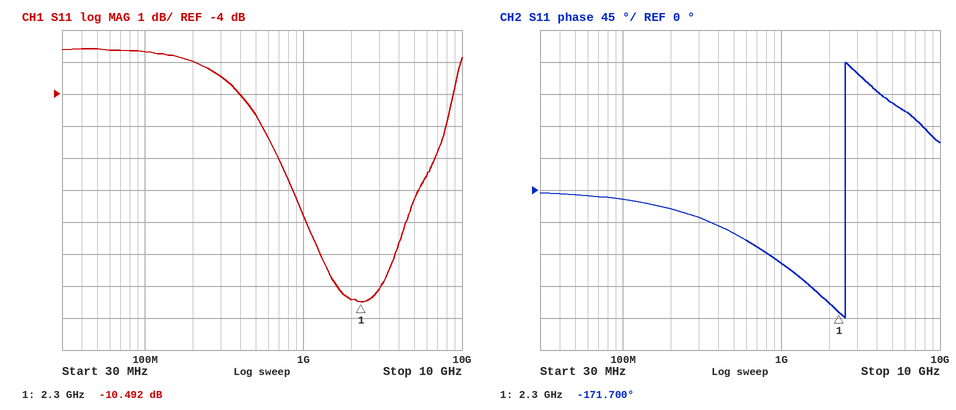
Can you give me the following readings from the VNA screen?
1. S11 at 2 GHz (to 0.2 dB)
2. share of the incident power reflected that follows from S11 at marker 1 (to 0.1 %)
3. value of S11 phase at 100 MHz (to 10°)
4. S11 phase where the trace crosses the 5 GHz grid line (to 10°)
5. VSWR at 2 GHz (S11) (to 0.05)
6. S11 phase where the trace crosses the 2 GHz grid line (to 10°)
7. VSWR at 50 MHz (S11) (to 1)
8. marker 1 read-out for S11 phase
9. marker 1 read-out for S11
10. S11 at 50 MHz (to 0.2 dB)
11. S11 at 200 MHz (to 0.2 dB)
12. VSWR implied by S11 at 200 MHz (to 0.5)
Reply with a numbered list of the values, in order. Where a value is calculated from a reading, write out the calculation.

1. -10.4 dB
2. 10^(-10.492/10) ≈ 8.9 %
3. -10°
4. 120°
5. |Γ| = 10^(-10.4/20) = 0.3020; VSWR = (1 + 0.3020)/(1 − 0.3020) ≈ 1.87, so 1.85 to the nearest 0.05
6. -160°
7. |Γ| = 10^(-2.6/20) = 0.7413; VSWR = (1 + 0.7413)/(1 − 0.7413) ≈ 7
8. -171.700°
9. -10.492 dB
10. -2.6 dB
11. -3.0 dB
12. |Γ| = 10^(-3/20) = 0.7079; VSWR = (1 + 0.7079)/(1 − 0.7079) ≈ 5.85, so 6.0 to the nearest 0.5
